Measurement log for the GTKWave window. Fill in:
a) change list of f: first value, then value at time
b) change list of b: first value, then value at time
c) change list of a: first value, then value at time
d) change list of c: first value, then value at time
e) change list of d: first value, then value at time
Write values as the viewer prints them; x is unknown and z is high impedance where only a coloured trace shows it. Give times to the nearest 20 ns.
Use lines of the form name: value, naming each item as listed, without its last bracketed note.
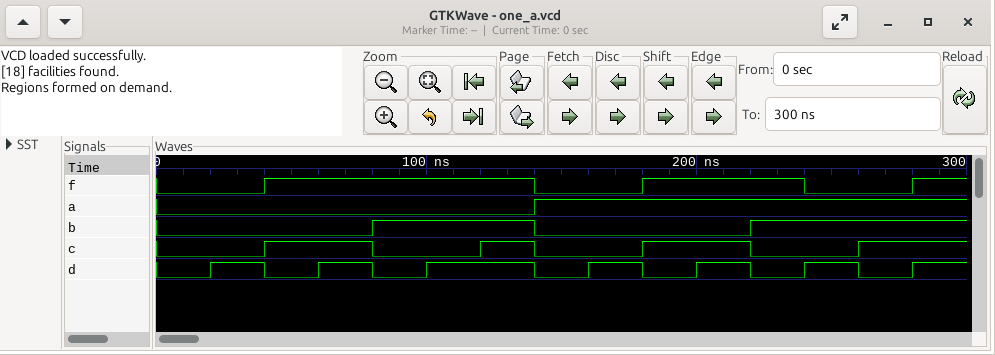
change list of f: first value, then value at time: 0, 1 at 40 ns, 0 at 140 ns, 1 at 180 ns, 0 at 240 ns, 1 at 280 ns
change list of b: first value, then value at time: 0, 1 at 80 ns, 0 at 140 ns, 1 at 220 ns
change list of a: first value, then value at time: 0, 1 at 140 ns
change list of c: first value, then value at time: 0, 1 at 40 ns, 0 at 80 ns, 1 at 120 ns, 0 at 140 ns, 1 at 180 ns, 0 at 220 ns, 1 at 260 ns
change list of d: first value, then value at time: 0, 1 at 20 ns, 0 at 40 ns, 1 at 60 ns, 0 at 80 ns, 1 at 100 ns, 0 at 140 ns, 1 at 160 ns, 0 at 180 ns, 1 at 200 ns, 0 at 220 ns, 1 at 240 ns, 0 at 260 ns, 1 at 280 ns
